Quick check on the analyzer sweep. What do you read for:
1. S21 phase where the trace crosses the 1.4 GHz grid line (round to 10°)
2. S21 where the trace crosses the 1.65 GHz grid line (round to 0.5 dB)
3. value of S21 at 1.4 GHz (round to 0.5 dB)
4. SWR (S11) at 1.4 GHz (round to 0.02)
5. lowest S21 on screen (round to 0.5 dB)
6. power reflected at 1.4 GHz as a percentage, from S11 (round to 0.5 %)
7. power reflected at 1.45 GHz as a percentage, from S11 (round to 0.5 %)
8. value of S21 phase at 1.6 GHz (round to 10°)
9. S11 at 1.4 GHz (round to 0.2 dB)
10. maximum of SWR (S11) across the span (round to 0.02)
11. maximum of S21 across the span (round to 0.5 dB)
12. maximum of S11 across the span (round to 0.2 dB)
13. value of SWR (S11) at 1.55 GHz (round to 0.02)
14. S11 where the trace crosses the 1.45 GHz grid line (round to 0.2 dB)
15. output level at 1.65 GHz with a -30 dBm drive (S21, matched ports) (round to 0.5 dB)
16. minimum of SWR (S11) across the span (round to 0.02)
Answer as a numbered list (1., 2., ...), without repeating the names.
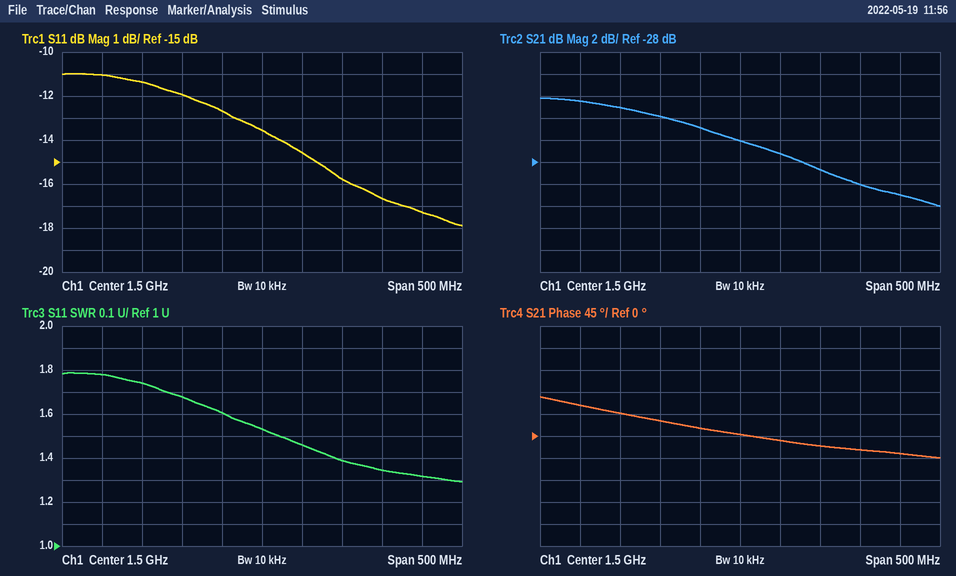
1. 30°
2. -30.0 dB
3. -24.0 dB
4. 1.68
5. -32.0 dB
6. 6.5 %
7. 5.5 %
8. -20°
9. -12.0 dB
10. 1.78
11. -22.0 dB
12. -11.0 dB
13. 1.46
14. -12.6 dB
15. -60.0 dBm
16. 1.30
